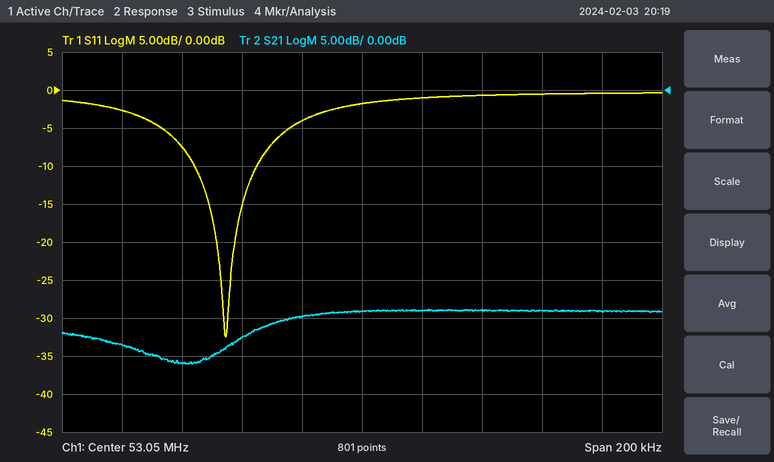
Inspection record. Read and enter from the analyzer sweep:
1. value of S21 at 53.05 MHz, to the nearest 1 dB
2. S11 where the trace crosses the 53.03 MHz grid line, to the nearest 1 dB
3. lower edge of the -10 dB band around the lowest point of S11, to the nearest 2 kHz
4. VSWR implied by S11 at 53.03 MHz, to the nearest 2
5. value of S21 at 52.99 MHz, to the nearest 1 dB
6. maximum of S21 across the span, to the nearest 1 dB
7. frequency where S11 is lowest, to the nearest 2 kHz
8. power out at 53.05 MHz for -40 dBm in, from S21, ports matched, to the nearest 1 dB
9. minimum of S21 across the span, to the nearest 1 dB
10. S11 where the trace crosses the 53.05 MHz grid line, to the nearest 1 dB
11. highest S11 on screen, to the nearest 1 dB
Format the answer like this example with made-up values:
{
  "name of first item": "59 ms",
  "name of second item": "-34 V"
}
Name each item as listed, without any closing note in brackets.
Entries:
{
  "value of S21 at 53.05 MHz, to the nearest 1 dB": "-29 dB",
  "S11 where the trace crosses the 53.03 MHz grid line, to the nearest 1 dB": "-4 dB",
  "lower edge of the -10 dB band around the lowest point of S11, to the nearest 2 kHz": "52.994 MHz",
  "VSWR implied by S11 at 53.03 MHz, to the nearest 2": "4",
  "value of S21 at 52.99 MHz, to the nearest 1 dB": "-36 dB",
  "maximum of S21 across the span, to the nearest 1 dB": "-29 dB",
  "frequency where S11 is lowest, to the nearest 2 kHz": "53.004 MHz",
  "power out at 53.05 MHz for -40 dBm in, from S21, ports matched, to the nearest 1 dB": "-69 dBm",
  "minimum of S21 across the span, to the nearest 1 dB": "-36 dB",
  "S11 where the trace crosses the 53.05 MHz grid line, to the nearest 1 dB": "-2 dB",
  "highest S11 on screen, to the nearest 1 dB": "0 dB"
}
